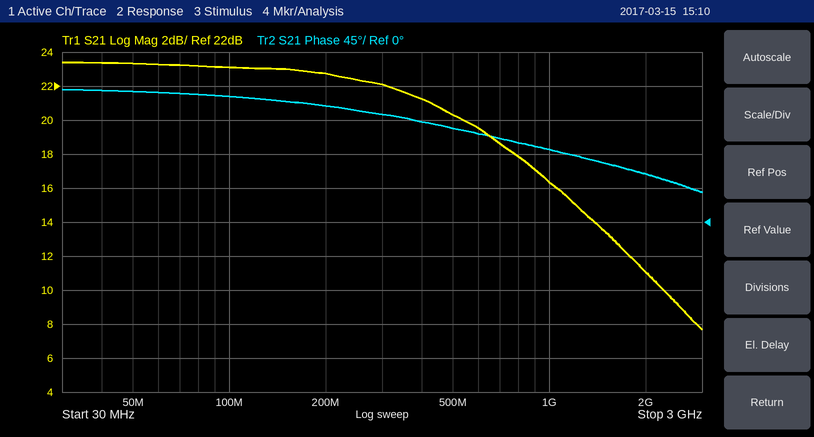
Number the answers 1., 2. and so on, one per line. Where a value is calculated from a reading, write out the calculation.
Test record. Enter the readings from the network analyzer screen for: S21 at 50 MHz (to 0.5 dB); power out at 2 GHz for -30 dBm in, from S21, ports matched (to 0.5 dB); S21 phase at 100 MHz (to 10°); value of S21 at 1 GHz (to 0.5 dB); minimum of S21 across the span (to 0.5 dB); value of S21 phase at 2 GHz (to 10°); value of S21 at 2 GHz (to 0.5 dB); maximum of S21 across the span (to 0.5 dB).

1. 23.5 dB
2. -30 dBm + (11.0 dB) = -19.0 dBm
3. 170°
4. 16.5 dB
5. 7.5 dB
6. 60°
7. 11.0 dB
8. 23.5 dB
